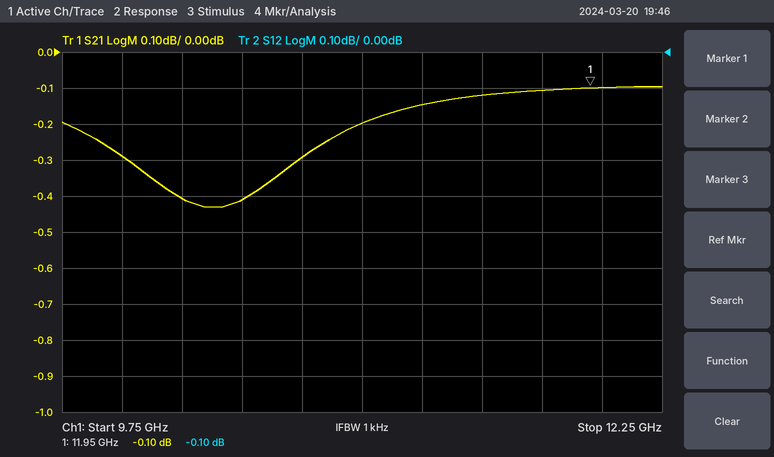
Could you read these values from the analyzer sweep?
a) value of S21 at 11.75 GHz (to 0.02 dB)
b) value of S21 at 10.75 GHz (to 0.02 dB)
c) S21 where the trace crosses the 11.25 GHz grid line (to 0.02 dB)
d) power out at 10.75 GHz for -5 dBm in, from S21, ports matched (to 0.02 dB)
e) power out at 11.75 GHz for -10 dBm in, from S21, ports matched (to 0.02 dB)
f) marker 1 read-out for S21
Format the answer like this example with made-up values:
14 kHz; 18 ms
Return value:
-0.10 dB; -0.30 dB; -0.14 dB; -5.30 dBm; -10.10 dBm; -0.10 dB
